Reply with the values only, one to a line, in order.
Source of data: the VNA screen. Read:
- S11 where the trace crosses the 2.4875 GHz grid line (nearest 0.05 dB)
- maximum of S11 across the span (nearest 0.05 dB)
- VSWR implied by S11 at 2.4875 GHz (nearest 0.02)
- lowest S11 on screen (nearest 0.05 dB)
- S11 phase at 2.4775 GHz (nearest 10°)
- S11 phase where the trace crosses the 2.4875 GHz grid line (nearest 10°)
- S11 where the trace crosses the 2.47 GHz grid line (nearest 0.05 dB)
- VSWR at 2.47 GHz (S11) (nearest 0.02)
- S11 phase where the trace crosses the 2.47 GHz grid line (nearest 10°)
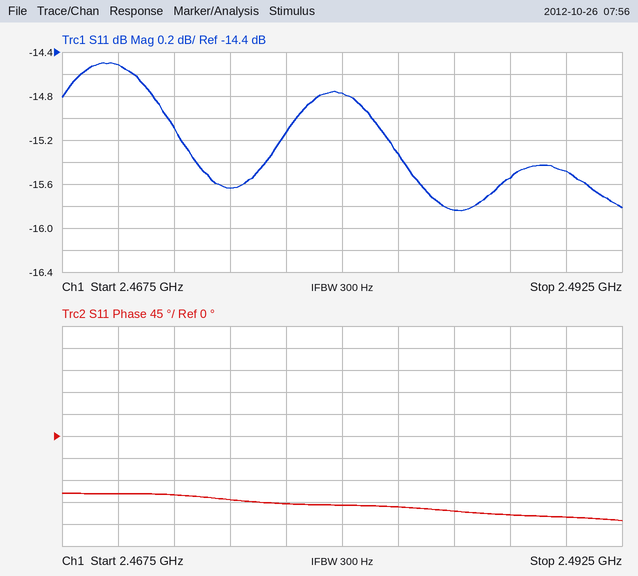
-15.55 dB
-14.50 dB
1.40
-15.85 dB
-140°
-160°
-14.50 dB
1.46
-120°
